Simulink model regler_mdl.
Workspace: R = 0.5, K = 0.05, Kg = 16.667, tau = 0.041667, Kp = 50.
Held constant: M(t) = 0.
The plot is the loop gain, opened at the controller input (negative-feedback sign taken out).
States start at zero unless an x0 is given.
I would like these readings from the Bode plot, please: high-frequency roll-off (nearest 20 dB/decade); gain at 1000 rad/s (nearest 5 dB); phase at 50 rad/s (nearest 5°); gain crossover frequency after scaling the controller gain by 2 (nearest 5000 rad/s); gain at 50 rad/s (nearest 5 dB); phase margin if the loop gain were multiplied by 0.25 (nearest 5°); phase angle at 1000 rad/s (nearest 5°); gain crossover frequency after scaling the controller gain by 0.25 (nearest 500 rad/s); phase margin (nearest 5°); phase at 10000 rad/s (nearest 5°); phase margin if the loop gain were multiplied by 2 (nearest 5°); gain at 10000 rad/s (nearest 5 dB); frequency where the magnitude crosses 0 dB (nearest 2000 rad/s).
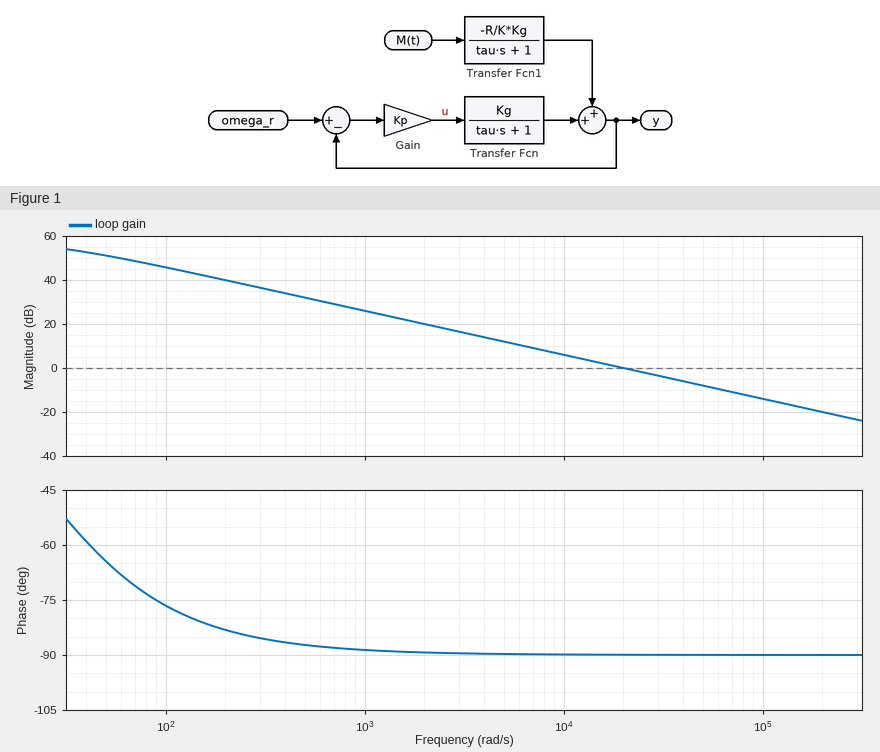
-20 dB/decade
25 dB
-65°
40000 rad/s
50 dB
90°
-90°
5000 rad/s
90°
-90°
90°
5 dB
20000 rad/s
